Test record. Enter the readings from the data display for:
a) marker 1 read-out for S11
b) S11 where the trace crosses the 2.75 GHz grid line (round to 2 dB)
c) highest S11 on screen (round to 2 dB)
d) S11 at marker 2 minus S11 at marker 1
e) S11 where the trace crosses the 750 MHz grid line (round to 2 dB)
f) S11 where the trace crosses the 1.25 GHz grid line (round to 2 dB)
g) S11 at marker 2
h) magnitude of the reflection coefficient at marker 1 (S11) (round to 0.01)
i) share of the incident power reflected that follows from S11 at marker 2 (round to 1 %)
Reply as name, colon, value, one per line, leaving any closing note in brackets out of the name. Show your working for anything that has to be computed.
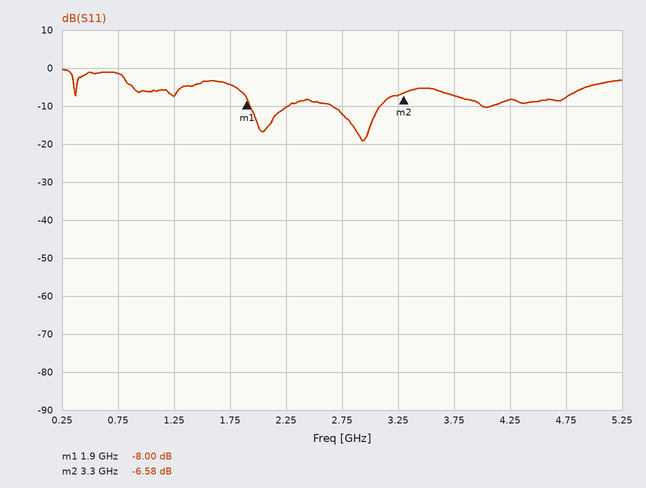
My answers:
marker 1 read-out for S11: -8.00 dB
S11 where the trace crosses the 2.75 GHz grid line: -12 dB
highest S11 on screen: 0 dB
S11 at marker 2 minus S11 at marker 1: -6.58 − (-8) = 1.42 dB
S11 where the trace crosses the 750 MHz grid line: -2 dB
S11 where the trace crosses the 1.25 GHz grid line: -8 dB
S11 at marker 2: -6.58 dB
magnitude of the reflection coefficient at marker 1 (S11): 10^(-8/20) ≈ 0.40
share of the incident power reflected that follows from S11 at marker 2: 10^(-6.58/10) ≈ 22 %
